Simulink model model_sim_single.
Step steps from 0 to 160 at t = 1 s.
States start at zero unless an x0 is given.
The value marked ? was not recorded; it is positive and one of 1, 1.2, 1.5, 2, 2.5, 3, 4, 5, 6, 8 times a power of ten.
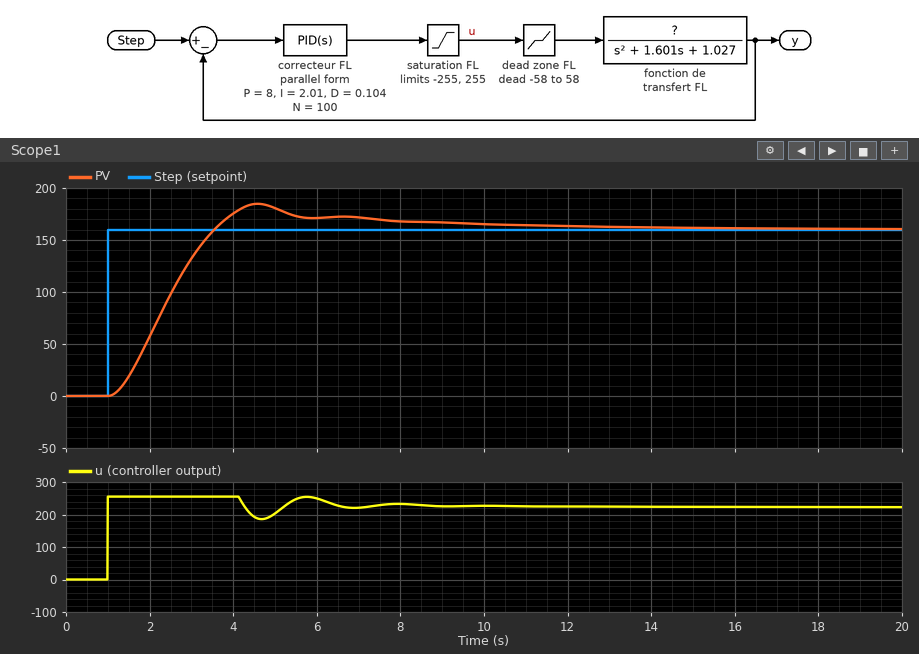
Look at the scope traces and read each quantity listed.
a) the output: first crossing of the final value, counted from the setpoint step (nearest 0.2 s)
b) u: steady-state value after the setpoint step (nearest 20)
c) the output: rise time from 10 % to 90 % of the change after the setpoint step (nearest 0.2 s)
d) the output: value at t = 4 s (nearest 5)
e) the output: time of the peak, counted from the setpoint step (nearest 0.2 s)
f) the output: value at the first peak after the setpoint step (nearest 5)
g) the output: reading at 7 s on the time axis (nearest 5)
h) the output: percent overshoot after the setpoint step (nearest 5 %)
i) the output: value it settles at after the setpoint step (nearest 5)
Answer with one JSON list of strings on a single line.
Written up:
["2.6 s", "220", "1.8 s", "175", "3.6 s", "185", "170", "15 %", "160"]
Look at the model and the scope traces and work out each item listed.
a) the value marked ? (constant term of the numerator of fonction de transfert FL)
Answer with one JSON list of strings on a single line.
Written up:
["1"]
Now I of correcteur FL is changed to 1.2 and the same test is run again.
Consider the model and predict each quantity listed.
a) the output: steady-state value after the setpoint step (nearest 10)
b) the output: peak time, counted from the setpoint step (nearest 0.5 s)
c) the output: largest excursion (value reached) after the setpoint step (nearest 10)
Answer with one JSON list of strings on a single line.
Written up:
["160", "3.0 s", "170"]
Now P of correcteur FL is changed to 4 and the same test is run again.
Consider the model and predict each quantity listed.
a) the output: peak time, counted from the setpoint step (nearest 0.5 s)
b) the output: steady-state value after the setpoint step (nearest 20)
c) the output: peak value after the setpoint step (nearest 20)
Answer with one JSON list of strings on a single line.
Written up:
["4.0 s", "160", "200"]
